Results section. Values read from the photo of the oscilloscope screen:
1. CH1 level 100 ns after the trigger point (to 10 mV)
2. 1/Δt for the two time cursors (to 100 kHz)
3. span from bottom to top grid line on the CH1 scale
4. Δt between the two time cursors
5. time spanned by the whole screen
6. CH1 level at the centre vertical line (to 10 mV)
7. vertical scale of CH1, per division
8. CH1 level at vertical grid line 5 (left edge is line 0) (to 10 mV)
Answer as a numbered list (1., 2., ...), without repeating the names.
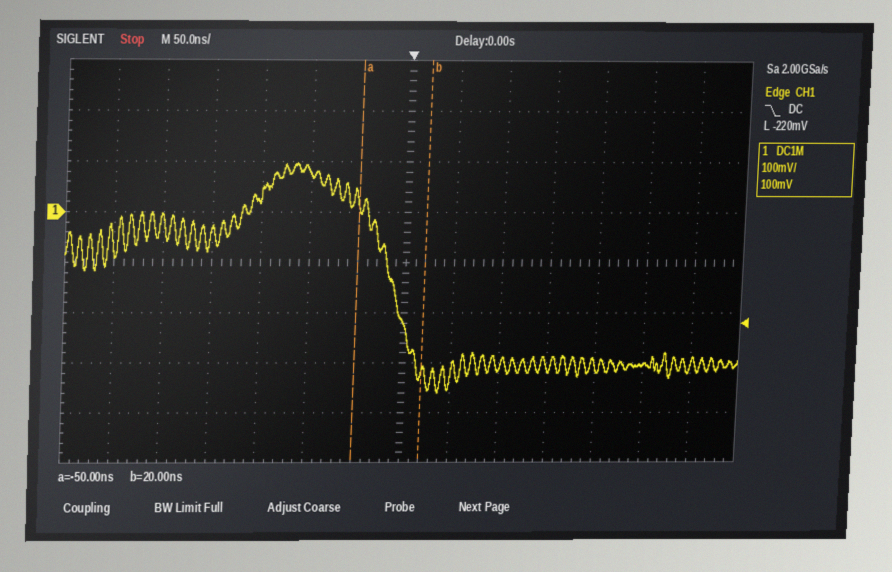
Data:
1. -310 mV
2. 14.3 MHz
3. 800 mV
4. 70 ns
5. 700 ns
6. -220 mV
7. 100 mV
8. 80 mV
